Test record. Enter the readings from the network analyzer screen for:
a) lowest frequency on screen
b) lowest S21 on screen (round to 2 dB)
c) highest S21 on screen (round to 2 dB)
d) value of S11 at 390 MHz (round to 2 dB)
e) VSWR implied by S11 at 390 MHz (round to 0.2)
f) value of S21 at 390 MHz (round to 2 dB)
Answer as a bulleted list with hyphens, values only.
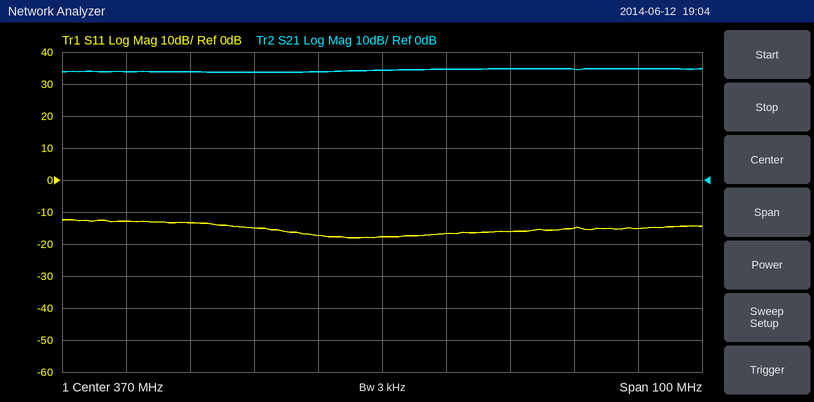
- 320 MHz
- 34 dB
- 34 dB
- -16 dB
- 1.4
- 34 dB
